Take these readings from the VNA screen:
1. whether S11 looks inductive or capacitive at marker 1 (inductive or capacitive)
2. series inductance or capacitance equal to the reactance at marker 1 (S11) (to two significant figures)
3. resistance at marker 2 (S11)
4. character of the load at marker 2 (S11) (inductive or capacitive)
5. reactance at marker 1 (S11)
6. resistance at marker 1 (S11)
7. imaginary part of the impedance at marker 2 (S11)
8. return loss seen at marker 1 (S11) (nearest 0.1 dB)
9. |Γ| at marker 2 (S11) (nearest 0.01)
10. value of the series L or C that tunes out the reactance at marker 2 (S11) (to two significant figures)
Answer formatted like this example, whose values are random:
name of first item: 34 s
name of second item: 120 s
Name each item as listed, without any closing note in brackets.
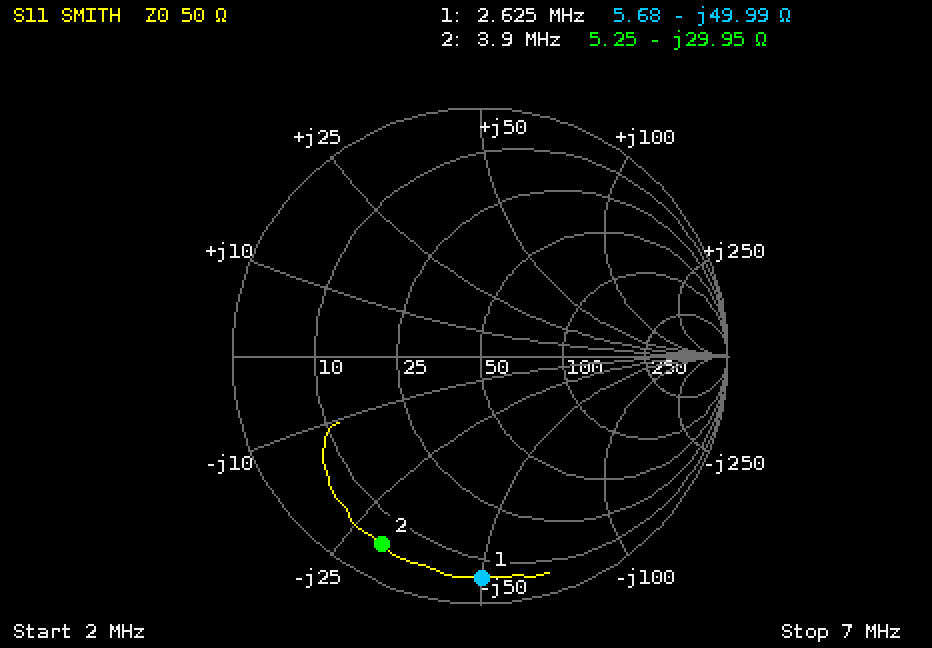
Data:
whether S11 looks inductive or capacitive at marker 1: capacitive
series inductance or capacitance equal to the reactance at marker 1 (S11): 1.2 nF
resistance at marker 2: 5.25 Ω
character of the load at marker 2 (S11): capacitive
reactance at marker 1: -49.99 Ω
resistance at marker 1: 5.68 Ω
imaginary part of the impedance at marker 2: -29.95 Ω
return loss seen at marker 1 (S11): 1.0 dB
|Γ| at marker 2 (S11): 0.86
value of the series L or C that tunes out the reactance at marker 2 (S11): 1.2 µH
